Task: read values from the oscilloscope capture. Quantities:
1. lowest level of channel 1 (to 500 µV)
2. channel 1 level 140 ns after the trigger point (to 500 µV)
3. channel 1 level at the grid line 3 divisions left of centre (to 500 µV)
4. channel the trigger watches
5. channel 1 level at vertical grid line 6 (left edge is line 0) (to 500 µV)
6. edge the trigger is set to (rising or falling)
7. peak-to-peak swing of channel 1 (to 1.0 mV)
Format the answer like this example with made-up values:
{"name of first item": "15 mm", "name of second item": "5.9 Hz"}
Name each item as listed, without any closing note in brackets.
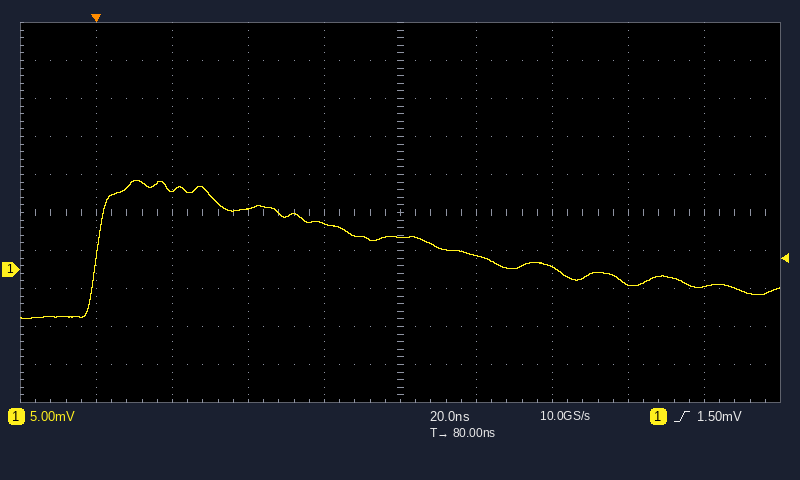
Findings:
{"lowest level of channel 1": "-6.5 mV", "channel 1 level 140 ns after the trigger point": "-2.0 mV", "channel 1 level at the grid line 3 divisions left of centre": "10.5 mV", "channel the trigger watches": "channel 1", "channel 1 level at vertical grid line 6 (left edge is line 0)": "2.0 mV", "edge the trigger is set to": "rising", "peak-to-peak swing of channel 1": "18.0 mV"}
